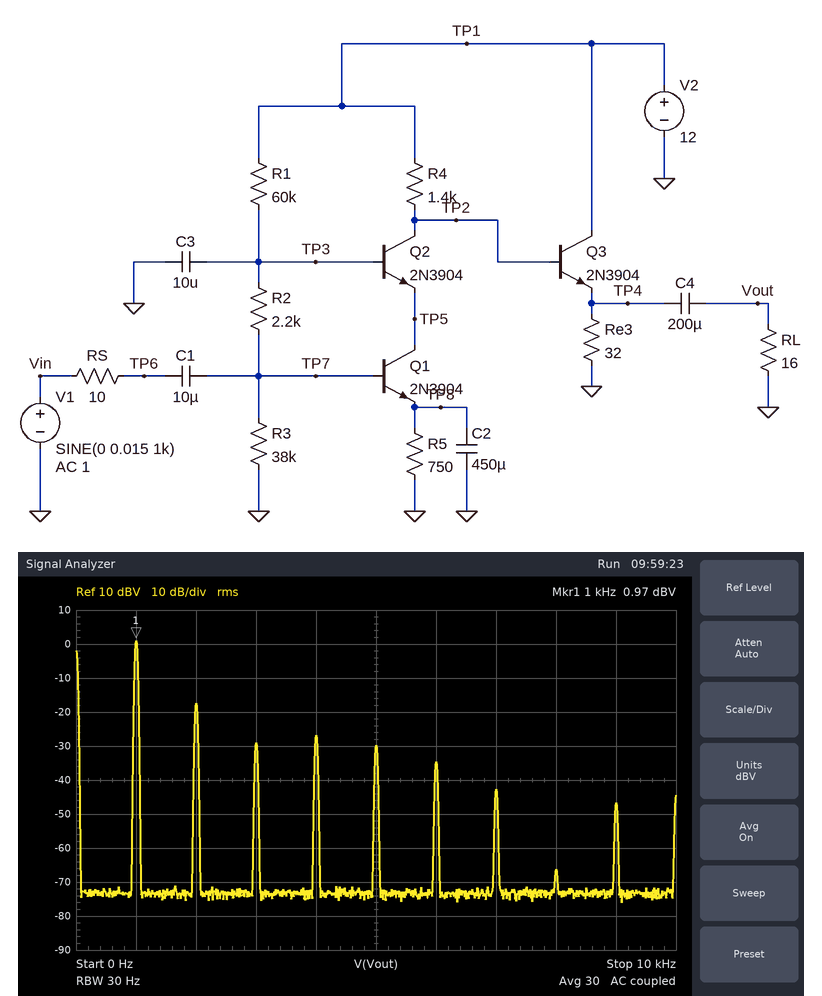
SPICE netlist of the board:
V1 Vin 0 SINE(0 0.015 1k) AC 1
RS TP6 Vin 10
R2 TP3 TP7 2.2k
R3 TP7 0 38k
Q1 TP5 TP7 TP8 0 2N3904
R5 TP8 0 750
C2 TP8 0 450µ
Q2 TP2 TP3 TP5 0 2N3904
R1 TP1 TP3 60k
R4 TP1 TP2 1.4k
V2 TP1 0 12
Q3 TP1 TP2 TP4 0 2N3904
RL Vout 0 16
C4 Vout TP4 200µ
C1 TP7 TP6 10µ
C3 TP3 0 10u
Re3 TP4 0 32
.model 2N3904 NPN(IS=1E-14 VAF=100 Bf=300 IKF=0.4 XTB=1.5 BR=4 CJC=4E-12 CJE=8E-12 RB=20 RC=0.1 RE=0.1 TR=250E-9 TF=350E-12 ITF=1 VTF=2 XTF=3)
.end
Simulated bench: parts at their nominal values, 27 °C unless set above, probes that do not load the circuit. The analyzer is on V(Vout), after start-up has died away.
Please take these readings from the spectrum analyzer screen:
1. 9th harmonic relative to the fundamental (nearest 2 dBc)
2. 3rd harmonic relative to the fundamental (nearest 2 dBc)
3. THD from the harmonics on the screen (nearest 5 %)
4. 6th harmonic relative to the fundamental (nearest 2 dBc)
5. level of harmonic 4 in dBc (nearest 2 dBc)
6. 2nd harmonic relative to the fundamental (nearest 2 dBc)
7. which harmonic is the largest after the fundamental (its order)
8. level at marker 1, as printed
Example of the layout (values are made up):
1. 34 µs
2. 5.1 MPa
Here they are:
1. -48 dBc
2. -30 dBc
3. 15 %
4. -36 dBc
5. -28 dBc
6. -18 dBc
7. 2
8. 0.97 dBV
